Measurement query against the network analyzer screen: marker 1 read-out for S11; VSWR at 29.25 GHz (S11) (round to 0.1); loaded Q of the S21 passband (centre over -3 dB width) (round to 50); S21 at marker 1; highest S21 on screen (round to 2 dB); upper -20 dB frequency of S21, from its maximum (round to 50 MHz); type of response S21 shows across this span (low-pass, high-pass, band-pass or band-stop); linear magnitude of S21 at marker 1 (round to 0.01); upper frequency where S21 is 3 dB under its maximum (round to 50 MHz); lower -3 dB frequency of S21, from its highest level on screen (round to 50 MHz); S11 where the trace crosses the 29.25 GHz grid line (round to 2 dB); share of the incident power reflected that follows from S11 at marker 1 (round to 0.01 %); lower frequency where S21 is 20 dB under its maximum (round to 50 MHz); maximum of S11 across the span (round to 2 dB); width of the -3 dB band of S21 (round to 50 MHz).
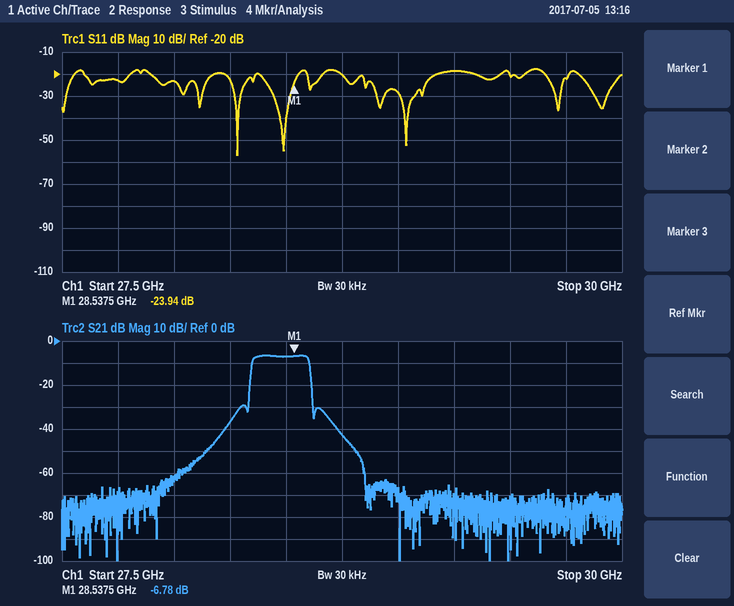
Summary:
-23.94 dB
1.3
100
-6.78 dB
-6 dB
28.60 GHz
band-pass
0.46
28.60 GHz
28.35 GHz
-18 dB
0.40 %
28.35 GHz
-18 dB
250 MHz
